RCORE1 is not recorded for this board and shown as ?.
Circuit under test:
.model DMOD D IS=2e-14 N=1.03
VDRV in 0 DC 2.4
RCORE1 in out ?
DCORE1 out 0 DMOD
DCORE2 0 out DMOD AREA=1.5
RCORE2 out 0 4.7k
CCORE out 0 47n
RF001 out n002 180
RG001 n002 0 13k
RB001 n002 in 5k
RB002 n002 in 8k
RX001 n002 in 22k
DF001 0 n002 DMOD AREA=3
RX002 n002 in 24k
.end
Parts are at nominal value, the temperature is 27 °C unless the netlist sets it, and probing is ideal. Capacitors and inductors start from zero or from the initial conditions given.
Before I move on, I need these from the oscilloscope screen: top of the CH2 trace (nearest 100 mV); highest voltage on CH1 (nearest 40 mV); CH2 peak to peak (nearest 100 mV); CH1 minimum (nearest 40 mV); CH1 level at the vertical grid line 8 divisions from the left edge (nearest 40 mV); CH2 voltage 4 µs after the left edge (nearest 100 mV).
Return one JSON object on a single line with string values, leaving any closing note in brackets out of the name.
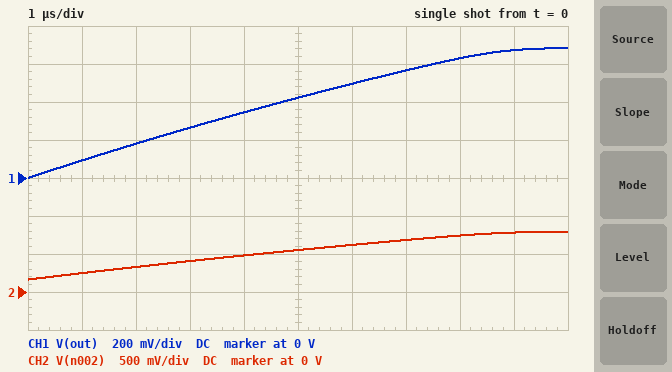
{"top of the CH2 trace": "800 mV", "highest voltage on CH1": "680 mV", "CH2 peak to peak": "600 mV", "CH1 minimum": "0 V", "CH1 level at the vertical grid line 8 divisions from the left edge": "640 mV", "CH2 voltage 4 µs after the left edge": "500 mV"}
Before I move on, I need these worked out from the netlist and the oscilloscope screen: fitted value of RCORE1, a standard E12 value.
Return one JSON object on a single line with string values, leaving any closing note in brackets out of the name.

{"fitted value of RCORE1, a standard E12 value": "680 Ω"}
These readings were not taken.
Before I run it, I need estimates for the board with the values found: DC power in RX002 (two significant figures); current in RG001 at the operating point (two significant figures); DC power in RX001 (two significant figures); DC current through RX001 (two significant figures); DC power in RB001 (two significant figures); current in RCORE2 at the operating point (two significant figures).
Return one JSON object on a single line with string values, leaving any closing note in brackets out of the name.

{"DC power in RX002": "110 µW", "current in RG001 at the operating point": "61 µA", "DC power in RX001": "120 µW", "DC current through RX001": "73 µA", "DC power in RB001": "520 µW", "current in RCORE2 at the operating point": "150 µA"}
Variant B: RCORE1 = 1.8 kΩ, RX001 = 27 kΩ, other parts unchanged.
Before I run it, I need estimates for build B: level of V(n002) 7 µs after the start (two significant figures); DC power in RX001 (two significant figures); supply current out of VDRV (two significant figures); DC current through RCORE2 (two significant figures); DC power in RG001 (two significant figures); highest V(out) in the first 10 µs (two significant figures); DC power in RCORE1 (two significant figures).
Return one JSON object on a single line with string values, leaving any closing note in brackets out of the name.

{"level of V(n002) 7 µs after the start": "440 mV", "DC power in RX001": "98 µW", "supply current out of VDRV": "1.6 mA", "DC current through RCORE2": "140 µA", "DC power in RG001": "46 µW", "highest V(out) in the first 10 µs": "420 mV", "DC power in RCORE1": "1.7 mW"}
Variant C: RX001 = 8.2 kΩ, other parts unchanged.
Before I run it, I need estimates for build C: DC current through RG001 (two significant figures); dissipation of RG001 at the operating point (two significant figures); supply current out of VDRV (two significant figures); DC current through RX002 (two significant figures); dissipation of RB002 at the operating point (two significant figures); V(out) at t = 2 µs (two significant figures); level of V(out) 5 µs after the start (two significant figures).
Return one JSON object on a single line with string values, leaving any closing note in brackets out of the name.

{"DC current through RG001": "63 µA", "dissipation of RG001 at the operating point": "51 µW", "supply current out of VDRV": "3.3 mA", "DC current through RX002": "66 µA", "dissipation of RB002 at the operating point": "310 µW", "V(out) at t = 2 µs": "190 mV", "level of V(out) 5 µs after the start": "440 mV"}
